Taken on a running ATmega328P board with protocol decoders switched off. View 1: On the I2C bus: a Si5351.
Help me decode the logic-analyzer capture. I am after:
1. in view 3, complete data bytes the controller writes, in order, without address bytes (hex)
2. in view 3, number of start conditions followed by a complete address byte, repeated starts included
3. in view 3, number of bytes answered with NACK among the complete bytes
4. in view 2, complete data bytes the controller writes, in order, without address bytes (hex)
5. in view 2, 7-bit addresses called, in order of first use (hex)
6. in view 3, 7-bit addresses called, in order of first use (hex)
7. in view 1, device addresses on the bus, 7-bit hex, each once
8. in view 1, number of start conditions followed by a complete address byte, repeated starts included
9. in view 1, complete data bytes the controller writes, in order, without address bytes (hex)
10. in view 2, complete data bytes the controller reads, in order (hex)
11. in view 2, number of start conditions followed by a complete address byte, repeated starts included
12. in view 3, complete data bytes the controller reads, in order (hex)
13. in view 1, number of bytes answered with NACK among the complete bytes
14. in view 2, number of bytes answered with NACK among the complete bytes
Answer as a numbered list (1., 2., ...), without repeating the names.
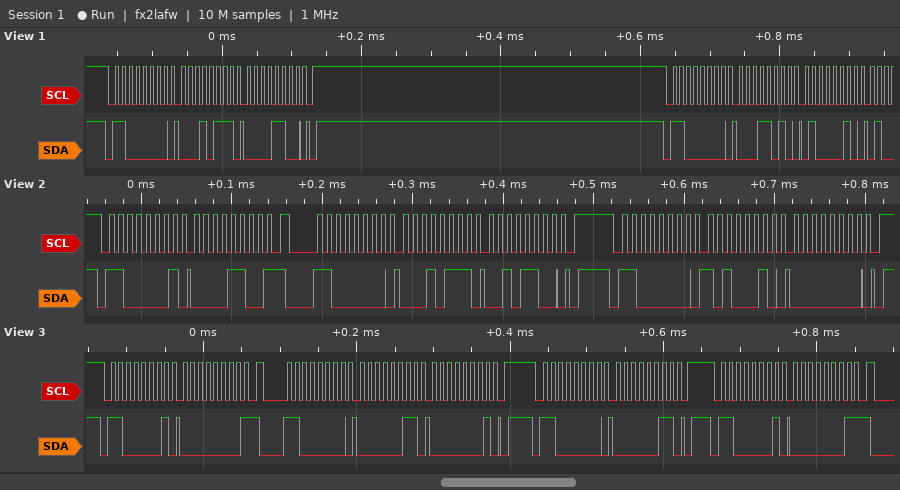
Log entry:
1. 03 01 03
2. 4
3. 2
4. 17 2C A2 00
5. 0x60
6. 0x60
7. 0x60
8. 2
9. 17 0C 1A 42
10. 0C
11. 3
12. 00 01
13. 0
14. 1
